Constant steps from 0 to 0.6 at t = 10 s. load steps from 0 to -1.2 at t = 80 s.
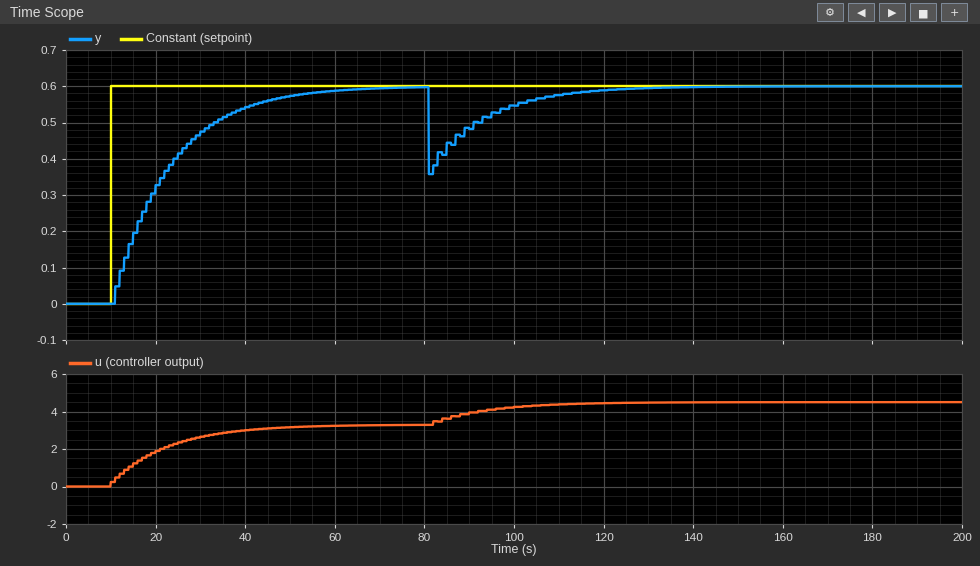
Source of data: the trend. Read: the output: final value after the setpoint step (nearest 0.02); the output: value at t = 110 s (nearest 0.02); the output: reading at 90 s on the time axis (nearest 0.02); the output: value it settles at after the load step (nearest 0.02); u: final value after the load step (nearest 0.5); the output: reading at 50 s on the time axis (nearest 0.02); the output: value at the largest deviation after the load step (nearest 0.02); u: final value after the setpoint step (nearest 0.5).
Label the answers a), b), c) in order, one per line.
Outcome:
a) 0.60
b) 0.58
c) 0.48
d) 0.60
e) 4.5
f) 0.58
g) 0.36
h) 3.5
